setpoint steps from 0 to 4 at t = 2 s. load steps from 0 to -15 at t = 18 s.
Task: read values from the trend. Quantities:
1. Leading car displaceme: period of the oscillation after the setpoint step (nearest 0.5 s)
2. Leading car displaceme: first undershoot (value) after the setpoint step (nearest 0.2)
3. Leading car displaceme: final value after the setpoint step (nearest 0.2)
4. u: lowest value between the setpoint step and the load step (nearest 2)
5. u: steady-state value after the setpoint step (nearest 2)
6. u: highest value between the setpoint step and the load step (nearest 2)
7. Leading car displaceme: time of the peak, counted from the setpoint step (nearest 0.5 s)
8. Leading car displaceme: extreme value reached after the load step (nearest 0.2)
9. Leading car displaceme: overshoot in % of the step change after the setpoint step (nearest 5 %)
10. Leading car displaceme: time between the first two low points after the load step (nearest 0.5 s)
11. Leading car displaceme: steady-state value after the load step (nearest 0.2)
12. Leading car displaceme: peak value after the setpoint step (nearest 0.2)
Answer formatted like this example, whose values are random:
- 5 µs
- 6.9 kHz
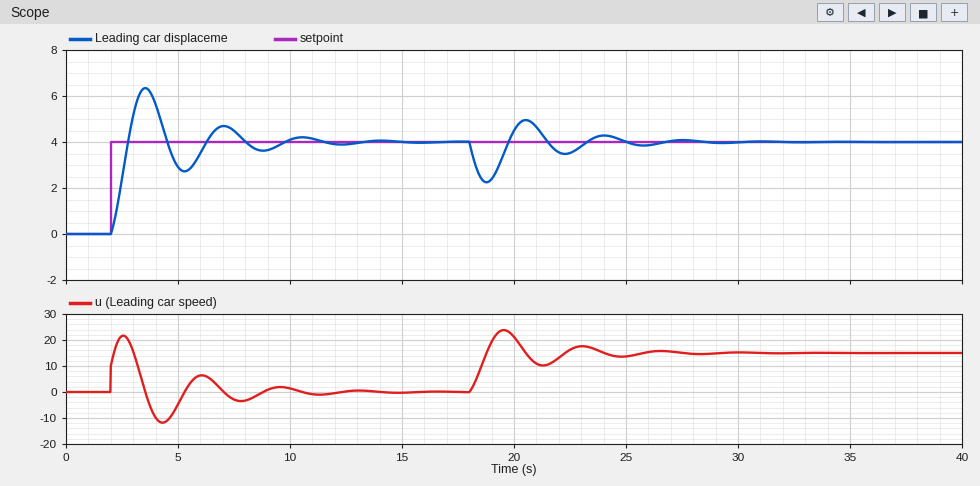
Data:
- 3.5 s
- 2.8
- 4.0
- -12
- 0
- 22
- 1.5 s
- 2.2
- 60 %
- 3.5 s
- 4.0
- 6.4
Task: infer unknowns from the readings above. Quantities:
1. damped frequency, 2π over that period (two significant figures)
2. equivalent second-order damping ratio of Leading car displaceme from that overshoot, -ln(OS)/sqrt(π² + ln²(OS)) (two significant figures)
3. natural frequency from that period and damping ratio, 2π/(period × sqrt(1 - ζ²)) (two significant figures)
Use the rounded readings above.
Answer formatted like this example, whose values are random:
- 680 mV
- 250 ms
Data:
- 1.8 rad/s
- 0.16
- 1.8 rad/s
